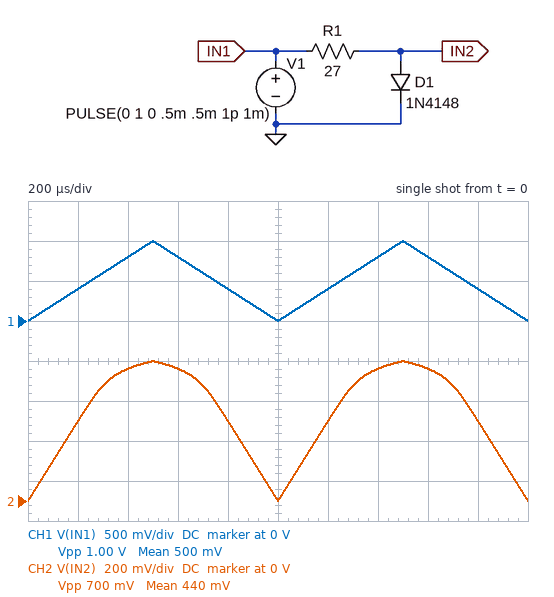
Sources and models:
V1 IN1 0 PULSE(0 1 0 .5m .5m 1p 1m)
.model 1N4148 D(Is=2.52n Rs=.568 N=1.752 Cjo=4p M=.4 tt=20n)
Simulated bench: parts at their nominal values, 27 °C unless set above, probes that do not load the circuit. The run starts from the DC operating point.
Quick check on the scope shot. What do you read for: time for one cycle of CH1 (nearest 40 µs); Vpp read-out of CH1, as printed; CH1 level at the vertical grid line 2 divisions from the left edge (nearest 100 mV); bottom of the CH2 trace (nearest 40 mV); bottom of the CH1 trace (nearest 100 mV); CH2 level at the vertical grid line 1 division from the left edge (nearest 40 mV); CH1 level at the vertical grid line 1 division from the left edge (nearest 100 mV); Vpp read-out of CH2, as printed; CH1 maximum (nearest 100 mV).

1.00 ms
1.00 V
800 mV
0 V
0 V
400 mV
400 mV
700 mV
1.0 V
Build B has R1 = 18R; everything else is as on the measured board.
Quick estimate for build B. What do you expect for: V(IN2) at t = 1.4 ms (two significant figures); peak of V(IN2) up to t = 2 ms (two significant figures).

680 mV
720 mV
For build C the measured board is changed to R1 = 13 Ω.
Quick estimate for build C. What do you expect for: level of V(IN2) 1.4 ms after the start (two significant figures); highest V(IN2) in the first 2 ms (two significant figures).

690 mV
730 mV
